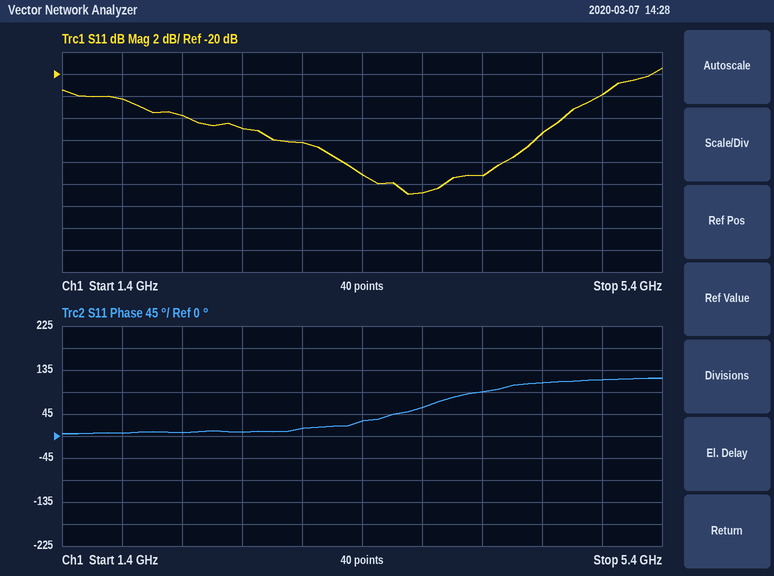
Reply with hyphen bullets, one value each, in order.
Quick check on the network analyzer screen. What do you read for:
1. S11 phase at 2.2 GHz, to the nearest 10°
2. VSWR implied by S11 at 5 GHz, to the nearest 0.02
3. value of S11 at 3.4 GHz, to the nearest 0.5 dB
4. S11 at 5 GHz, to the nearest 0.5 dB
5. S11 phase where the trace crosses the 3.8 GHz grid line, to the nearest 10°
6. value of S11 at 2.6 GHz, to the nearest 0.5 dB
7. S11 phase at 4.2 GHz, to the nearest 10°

- 10°
- 1.18
- -29.0 dB
- -22.0 dB
- 60°
- -25.0 dB
- 90°
